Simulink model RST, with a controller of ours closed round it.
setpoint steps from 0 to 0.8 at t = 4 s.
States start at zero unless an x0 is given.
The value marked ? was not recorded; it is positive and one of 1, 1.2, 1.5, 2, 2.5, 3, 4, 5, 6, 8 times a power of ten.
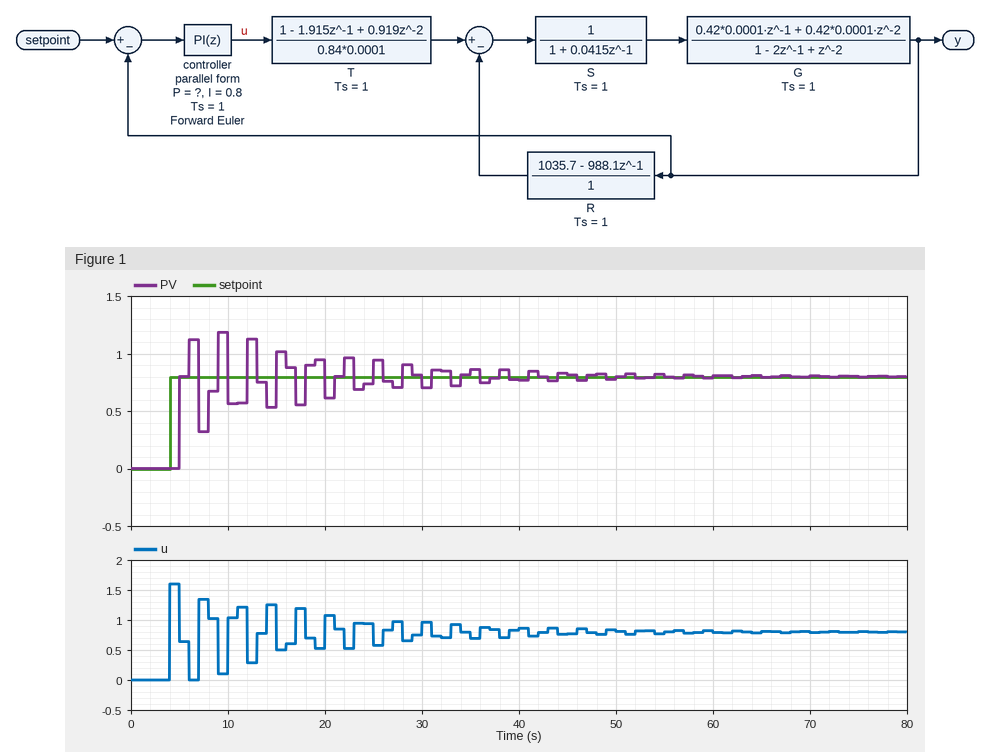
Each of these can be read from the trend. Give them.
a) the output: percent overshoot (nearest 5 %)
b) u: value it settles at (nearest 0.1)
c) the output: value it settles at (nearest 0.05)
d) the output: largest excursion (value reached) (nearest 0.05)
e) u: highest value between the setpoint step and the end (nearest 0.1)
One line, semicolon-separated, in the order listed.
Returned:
50 %; 0.8; 0.80; 1.20; 1.6
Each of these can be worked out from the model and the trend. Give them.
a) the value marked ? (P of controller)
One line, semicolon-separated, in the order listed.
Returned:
2
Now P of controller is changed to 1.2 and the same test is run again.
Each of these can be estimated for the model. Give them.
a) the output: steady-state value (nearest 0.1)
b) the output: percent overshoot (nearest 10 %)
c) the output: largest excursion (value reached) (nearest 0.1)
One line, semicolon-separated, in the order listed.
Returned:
0.8; 20 %; 1.0
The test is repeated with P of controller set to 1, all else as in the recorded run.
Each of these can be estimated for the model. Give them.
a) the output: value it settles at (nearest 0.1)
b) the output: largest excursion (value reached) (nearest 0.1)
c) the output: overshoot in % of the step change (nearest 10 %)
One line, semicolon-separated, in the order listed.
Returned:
0.8; 0.9; 20 %
